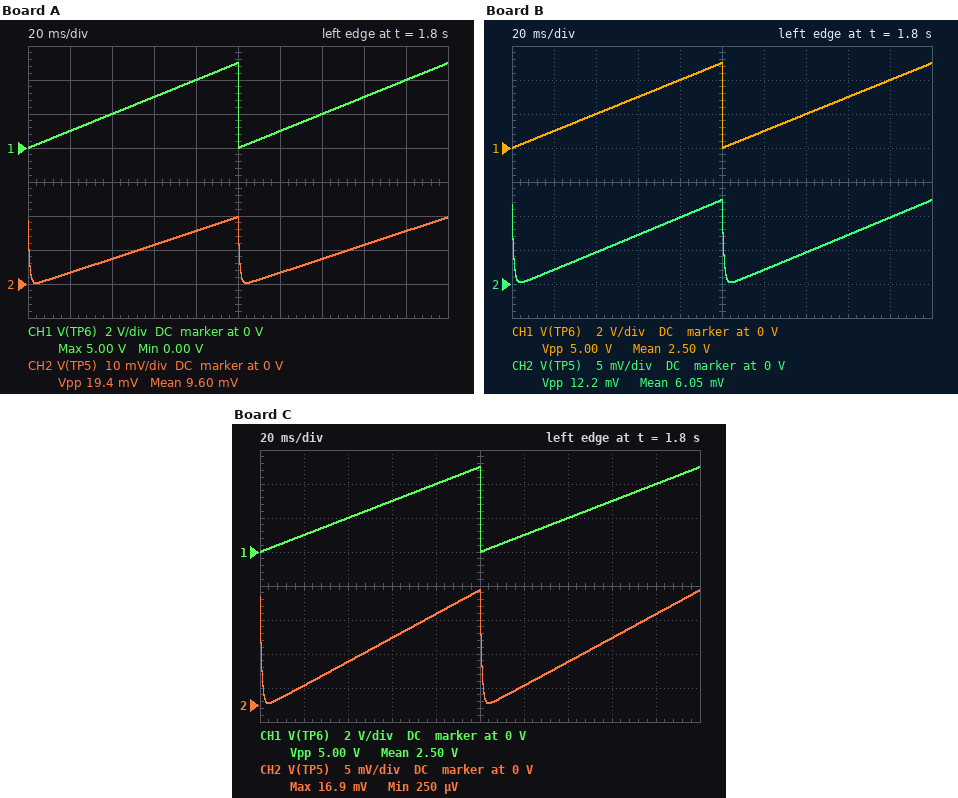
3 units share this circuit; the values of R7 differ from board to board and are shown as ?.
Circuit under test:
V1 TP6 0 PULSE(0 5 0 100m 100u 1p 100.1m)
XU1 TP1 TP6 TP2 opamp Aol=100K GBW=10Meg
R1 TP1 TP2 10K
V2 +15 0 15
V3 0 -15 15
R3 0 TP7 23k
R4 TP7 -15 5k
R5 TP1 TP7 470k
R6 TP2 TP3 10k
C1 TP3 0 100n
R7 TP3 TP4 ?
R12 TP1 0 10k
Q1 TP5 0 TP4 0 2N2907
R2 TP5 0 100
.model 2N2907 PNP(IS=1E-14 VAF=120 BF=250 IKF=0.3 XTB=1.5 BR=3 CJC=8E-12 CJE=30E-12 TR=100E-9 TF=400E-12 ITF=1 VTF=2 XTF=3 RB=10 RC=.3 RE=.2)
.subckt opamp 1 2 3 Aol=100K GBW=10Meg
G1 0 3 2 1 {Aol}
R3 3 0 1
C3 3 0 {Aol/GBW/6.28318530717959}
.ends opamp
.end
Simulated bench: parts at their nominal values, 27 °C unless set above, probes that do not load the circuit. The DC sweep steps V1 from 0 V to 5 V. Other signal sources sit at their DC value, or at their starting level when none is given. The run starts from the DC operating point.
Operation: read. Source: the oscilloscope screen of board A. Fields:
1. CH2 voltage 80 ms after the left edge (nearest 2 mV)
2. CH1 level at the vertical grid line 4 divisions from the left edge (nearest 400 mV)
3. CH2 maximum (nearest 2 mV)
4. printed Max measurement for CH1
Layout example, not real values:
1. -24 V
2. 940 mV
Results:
1. 16 mV
2. 4.0 V
3. 20 mV
4. 5.00 V
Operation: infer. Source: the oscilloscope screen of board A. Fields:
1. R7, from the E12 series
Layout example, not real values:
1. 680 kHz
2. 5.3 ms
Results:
1. 39 kΩ
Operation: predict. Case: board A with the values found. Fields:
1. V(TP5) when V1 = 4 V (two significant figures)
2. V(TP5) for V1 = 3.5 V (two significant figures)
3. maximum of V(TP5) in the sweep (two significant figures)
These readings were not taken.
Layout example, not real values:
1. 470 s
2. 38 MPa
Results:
1. 16 mV
2. 14 mV
3. 20 mV
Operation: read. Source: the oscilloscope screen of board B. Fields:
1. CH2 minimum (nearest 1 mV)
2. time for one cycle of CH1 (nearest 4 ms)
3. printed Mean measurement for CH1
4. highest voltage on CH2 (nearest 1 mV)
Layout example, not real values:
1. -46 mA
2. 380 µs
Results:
1. 0 V
2. 100 ms
3. 2.50 V
4. 12 mV
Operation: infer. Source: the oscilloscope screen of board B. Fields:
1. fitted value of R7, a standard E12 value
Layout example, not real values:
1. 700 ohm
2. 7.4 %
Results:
1. 68 kΩ
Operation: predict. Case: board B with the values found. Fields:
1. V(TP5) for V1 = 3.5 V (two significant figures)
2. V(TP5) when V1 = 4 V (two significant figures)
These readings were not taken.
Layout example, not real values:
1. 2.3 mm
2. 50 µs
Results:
1. 8.6 mV
2. 9.9 mV
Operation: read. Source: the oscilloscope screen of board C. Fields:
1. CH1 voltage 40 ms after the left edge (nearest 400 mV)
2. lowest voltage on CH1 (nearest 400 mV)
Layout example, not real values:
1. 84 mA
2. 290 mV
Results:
1. 2.0 V
2. 0 V
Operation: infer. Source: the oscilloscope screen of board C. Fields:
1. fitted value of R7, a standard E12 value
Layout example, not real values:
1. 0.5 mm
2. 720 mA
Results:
1. 47 kΩ
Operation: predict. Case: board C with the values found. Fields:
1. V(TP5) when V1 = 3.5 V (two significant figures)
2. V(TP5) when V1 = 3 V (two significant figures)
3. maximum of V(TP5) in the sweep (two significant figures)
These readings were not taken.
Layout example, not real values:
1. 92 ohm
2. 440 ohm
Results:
1. 12 mV
2. 10 mV
3. 17 mV
